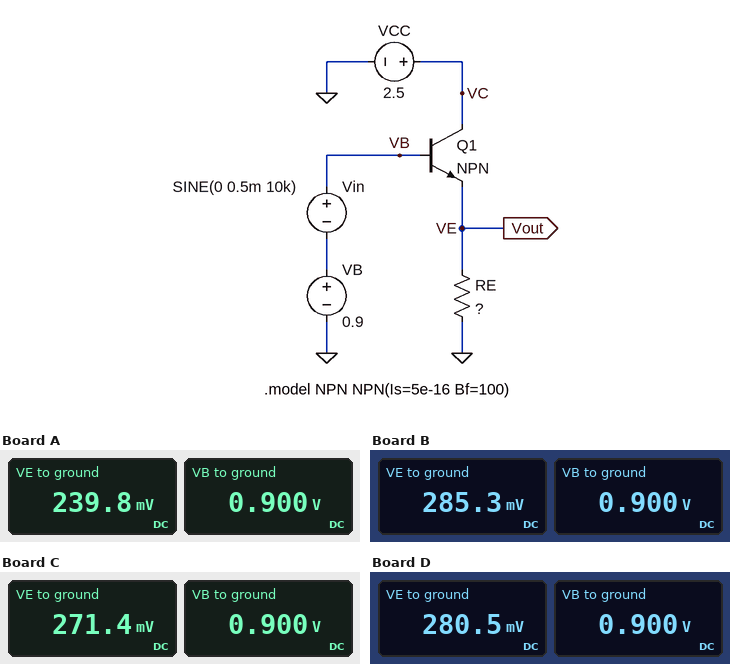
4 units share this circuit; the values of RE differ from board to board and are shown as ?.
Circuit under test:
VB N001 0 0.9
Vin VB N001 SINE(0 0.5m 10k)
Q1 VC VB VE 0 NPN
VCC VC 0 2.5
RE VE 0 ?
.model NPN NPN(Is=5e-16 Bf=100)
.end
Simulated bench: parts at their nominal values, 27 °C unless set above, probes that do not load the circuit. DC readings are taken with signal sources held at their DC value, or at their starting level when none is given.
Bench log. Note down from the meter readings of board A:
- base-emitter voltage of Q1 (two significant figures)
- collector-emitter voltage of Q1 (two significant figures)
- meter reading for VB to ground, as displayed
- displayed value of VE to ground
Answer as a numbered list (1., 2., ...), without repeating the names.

1. 660 mV
2. 2.3 V
3. 0.900 V
4. 239.8 mV
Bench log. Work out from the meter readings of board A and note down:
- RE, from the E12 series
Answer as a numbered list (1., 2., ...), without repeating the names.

1. 3.9 kΩ
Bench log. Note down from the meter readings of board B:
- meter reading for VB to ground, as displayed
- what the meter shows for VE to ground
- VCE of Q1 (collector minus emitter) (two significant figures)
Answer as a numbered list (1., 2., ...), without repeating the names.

1. 0.900 V
2. 285.3 mV
3. 2.2 V
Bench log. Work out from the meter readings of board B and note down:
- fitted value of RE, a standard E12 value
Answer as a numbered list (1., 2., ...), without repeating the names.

1. 27 kΩ
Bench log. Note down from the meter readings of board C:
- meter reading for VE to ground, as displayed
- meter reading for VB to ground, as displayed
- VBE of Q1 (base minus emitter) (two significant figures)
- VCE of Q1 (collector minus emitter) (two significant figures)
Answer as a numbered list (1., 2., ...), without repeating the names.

1. 271.4 mV
2. 0.900 V
3. 630 mV
4. 2.2 V
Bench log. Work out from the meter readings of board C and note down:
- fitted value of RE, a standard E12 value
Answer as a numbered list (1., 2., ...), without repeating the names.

1. 15 kΩ
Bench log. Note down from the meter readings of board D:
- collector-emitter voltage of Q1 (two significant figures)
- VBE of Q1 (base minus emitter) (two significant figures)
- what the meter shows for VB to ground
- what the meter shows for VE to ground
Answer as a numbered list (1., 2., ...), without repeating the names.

1. 2.2 V
2. 620 mV
3. 0.900 V
4. 280.5 mV
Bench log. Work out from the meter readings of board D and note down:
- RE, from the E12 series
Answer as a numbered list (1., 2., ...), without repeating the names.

1. 22 kΩ
